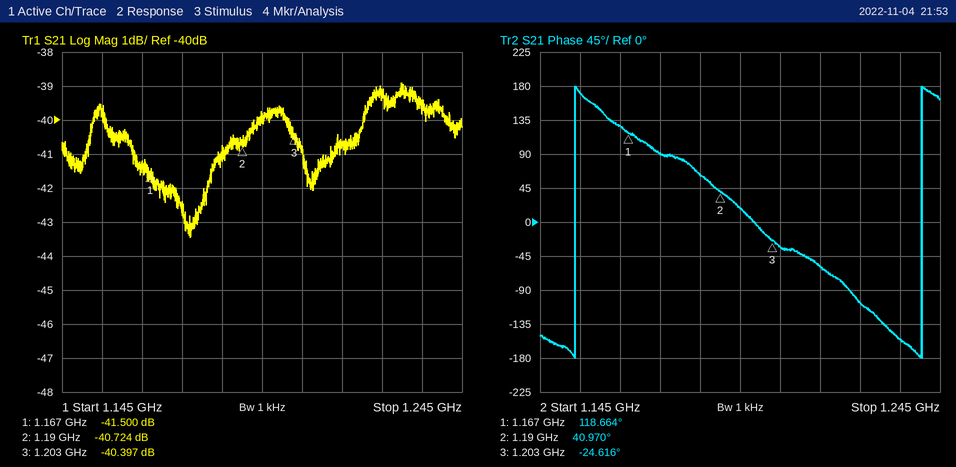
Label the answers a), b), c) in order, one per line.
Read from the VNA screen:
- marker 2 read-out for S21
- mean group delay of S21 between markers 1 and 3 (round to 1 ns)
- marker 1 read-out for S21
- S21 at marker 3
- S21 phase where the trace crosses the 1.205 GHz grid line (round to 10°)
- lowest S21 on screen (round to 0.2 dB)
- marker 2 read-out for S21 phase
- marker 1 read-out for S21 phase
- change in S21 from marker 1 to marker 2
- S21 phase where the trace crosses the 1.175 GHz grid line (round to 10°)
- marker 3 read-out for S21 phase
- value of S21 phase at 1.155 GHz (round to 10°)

a) -40.724 dB
b) 11 ns
c) -41.500 dB
d) -40.397 dB
e) -30°
f) -43.4 dB
g) 40.970°
h) 118.664°
i) 0.776 dB
j) 90°
k) -24.616°
l) 170°
